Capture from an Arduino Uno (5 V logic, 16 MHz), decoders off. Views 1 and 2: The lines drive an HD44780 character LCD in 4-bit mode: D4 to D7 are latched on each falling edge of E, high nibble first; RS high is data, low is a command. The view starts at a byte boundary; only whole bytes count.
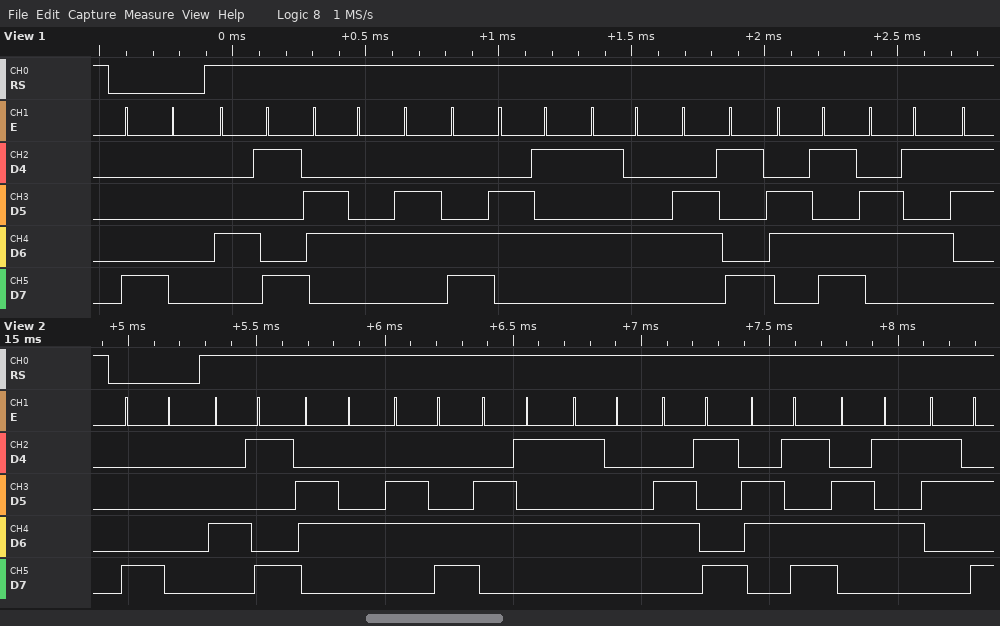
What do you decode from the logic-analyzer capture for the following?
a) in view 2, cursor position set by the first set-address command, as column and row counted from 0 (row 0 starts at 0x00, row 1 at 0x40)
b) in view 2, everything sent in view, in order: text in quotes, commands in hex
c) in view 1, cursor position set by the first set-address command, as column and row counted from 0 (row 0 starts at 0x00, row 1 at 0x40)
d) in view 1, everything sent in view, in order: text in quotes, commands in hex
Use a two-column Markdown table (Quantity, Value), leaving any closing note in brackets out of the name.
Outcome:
| Quantity | Value |
|---|---|
| in view 2, cursor position set by the first set-address command, as column and row counted from 0 | column 0, row 0 |
| in view 2, everything sent in view, in order: text in quotes, commands in hex | 0x80 "IdleTime:" |
| in view 1, cursor position set by the first set-address command, as column and row counted from 0 | column 0, row 0 |
| in view 1, everything sent in view, in order: text in quotes, commands in hex | 0x80 "IdleTime" |
